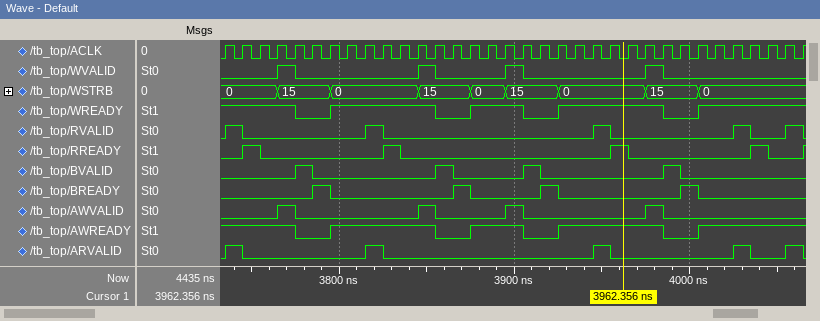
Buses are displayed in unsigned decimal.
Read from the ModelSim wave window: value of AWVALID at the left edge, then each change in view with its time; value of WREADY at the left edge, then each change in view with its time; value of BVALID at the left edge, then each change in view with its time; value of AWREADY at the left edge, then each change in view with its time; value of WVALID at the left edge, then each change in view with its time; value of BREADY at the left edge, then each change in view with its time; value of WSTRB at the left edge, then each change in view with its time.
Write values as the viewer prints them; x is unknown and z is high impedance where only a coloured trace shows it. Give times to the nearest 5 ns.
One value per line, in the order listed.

0, 1 at 3765 ns, 0 at 3775 ns, 1 at 3845 ns, 0 at 3855 ns, 1 at 3895 ns, 0 at 3905 ns, 1 at 3975 ns, 0 at 3985 ns
1, 0 at 3775 ns, 1 at 3795 ns, 0 at 3855 ns, 1 at 3875 ns, 0 at 3905 ns, 1 at 3925 ns, 0 at 3985 ns, 1 at 4005 ns
0, 1 at 3775 ns, 0 at 3785 ns, 1 at 3855 ns, 0 at 3865 ns, 1 at 3905 ns, 0 at 3915 ns, 1 at 3985 ns, 0 at 3995 ns
1, 0 at 3775 ns, 1 at 3795 ns, 0 at 3855 ns, 1 at 3875 ns, 0 at 3905 ns, 1 at 3925 ns, 0 at 3985 ns, 1 at 4005 ns
0, 1 at 3765 ns, 0 at 3775 ns, 1 at 3845 ns, 0 at 3855 ns, 1 at 3895 ns, 0 at 3905 ns, 1 at 3975 ns, 0 at 3985 ns
0, 1 at 3785 ns, 0 at 3795 ns, 1 at 3865 ns, 0 at 3875 ns, 1 at 3915 ns, 0 at 3925 ns, 1 at 3995 ns, 0 at 4005 ns
0, 15 at 3765 ns, 0 at 3795 ns, 15 at 3845 ns, 0 at 3875 ns, 15 at 3895 ns, 0 at 3925 ns, 15 at 3975 ns, 0 at 4005 ns
